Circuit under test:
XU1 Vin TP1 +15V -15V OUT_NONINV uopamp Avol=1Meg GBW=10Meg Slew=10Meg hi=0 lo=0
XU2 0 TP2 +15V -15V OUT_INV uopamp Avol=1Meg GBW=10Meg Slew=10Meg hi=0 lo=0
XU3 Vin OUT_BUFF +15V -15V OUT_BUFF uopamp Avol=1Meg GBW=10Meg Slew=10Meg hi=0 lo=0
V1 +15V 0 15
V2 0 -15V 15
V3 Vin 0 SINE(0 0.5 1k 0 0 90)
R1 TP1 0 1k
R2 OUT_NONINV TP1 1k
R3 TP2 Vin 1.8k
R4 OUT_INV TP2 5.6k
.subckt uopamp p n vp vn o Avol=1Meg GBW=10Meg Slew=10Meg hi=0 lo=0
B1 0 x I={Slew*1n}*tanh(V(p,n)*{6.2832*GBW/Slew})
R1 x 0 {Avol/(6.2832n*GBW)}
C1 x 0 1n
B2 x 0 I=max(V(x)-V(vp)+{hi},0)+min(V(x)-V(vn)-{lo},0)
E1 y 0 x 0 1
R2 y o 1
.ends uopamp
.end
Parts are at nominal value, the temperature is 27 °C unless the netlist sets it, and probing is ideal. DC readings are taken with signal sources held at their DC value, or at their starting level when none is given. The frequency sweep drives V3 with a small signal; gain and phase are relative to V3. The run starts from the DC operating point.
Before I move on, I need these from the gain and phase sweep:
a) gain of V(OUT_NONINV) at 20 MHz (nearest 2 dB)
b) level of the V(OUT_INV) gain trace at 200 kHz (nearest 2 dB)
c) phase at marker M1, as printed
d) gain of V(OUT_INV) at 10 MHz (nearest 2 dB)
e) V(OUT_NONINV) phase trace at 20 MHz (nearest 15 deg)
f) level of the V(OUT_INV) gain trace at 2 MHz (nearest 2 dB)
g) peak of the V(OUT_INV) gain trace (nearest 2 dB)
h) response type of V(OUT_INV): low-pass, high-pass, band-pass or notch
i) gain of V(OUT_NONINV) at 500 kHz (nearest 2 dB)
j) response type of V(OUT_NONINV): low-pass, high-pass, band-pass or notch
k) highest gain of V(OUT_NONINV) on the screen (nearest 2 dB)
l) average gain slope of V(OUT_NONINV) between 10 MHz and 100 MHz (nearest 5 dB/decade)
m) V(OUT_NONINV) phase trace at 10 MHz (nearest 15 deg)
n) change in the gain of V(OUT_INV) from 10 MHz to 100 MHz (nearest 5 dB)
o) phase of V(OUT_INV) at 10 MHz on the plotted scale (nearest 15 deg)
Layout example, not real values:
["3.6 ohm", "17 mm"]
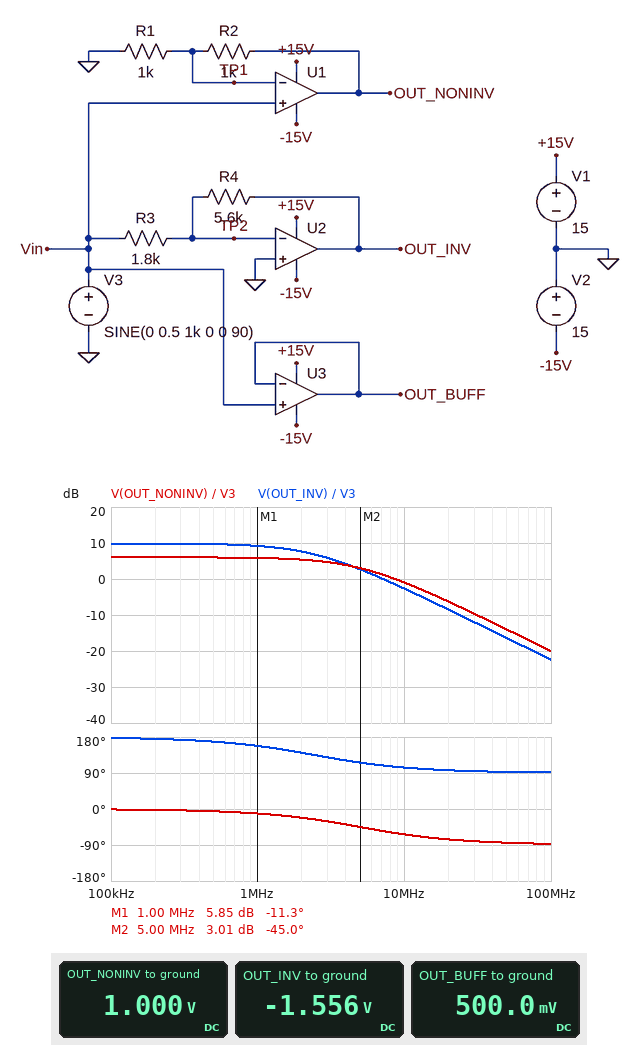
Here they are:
["-6 dB", "10 dB", "-11.3 deg", "-2 dB", "-75 deg", "8 dB", "10 dB", "low-pass", "6 dB", "low-pass", "6 dB", "-20 dB/decade", "-60 deg", "-20 dB", "105 deg"]
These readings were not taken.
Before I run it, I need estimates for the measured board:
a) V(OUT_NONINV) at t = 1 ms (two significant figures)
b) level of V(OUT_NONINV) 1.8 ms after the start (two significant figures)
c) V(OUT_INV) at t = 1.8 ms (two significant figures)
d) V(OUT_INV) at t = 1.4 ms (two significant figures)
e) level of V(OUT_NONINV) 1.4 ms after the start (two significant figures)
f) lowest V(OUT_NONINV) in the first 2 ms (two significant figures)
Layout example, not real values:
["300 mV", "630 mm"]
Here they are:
["1.0 V", "310 mV", "-480 mV", "1.3 V", "-810 mV", "-1.0 V"]
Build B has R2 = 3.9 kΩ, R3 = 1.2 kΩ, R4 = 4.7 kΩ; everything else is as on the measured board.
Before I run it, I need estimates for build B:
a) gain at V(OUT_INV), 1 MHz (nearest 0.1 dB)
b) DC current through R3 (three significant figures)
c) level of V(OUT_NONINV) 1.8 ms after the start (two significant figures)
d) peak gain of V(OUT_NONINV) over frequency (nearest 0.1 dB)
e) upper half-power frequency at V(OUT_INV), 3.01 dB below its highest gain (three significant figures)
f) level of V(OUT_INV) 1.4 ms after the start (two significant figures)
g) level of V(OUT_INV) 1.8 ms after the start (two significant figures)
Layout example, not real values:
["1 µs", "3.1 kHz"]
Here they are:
["10.9 dB", "417 µA", "760 mV", "13.8 dB", "2.03 MHz", "1.6 V", "-600 mV"]
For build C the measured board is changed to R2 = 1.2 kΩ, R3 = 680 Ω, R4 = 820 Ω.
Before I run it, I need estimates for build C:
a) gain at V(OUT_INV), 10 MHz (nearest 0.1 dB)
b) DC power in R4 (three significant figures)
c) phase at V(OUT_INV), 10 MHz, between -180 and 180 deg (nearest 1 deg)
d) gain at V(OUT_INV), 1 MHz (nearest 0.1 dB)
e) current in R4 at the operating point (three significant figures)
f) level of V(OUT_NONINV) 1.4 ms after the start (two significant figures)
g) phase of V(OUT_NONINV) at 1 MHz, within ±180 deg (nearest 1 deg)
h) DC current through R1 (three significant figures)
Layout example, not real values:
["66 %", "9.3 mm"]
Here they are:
["-6.1 dB", "443 µW", "114 deg", "1.4 dB", "735 µA", "-890 mV", "-12 deg", "500 µA"]
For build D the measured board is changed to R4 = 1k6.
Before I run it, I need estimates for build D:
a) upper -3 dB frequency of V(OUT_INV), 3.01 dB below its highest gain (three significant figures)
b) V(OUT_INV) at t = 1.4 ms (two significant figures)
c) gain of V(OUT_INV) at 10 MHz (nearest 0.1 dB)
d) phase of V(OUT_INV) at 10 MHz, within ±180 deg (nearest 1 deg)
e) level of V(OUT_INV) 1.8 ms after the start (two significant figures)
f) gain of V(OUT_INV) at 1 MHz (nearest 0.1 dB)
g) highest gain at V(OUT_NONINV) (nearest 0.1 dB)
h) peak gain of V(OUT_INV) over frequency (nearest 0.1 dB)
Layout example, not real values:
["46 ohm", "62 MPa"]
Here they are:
["5.29 MHz", "360 mV", "-7.6 dB", "118 deg", "-140 mV", "-1.2 dB", "6.0 dB", "-1.0 dB"]
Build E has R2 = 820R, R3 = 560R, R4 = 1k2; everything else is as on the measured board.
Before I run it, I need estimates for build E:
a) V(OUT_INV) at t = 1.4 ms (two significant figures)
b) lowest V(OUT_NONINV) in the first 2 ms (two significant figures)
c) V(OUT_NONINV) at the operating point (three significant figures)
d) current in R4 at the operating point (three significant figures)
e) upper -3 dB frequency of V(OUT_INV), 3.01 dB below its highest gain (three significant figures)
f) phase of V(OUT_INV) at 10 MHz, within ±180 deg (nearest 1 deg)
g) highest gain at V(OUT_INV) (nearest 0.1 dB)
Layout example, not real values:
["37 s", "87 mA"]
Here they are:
["870 mV", "-910 mV", "910 mV", "893 µA", "3.18 MHz", "108 deg", "6.6 dB"]
